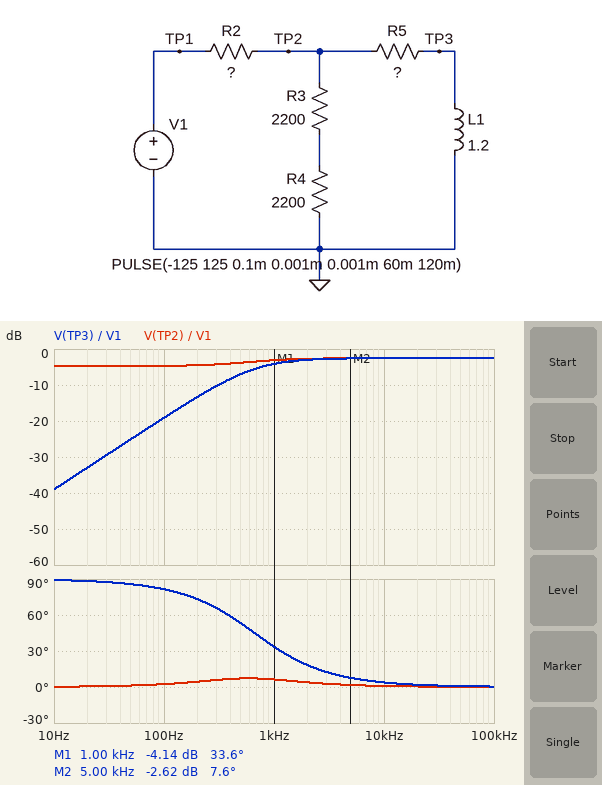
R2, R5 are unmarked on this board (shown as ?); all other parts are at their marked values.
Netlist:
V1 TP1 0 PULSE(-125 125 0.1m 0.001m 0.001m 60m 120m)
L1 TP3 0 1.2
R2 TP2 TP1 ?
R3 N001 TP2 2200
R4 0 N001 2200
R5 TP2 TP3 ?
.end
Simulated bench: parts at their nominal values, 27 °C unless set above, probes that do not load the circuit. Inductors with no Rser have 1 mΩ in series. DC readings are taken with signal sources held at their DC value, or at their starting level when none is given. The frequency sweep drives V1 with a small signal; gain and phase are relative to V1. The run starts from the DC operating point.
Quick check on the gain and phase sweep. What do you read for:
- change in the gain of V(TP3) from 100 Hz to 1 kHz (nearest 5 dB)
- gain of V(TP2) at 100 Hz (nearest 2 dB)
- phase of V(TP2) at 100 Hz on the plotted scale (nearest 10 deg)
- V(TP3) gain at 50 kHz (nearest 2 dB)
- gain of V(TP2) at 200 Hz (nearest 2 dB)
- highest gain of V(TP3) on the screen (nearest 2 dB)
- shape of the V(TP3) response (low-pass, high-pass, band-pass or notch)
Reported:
15 dB
-4 dB
0 deg
-2 dB
-4 dB
-2 dB
high-pass
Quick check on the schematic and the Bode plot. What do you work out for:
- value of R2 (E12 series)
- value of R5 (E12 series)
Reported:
1.5 kΩ
3.9 kΩ
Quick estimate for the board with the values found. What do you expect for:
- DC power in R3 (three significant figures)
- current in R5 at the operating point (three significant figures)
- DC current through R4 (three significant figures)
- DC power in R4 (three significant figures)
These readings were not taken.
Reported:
596 mW
18.6 mA
16.5 mA
596 mW
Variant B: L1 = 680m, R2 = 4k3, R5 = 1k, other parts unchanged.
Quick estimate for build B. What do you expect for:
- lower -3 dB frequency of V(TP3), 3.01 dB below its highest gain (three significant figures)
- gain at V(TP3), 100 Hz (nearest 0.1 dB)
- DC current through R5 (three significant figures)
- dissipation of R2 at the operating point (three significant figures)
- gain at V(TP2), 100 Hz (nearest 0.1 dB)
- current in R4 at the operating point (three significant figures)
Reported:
743 Hz
-23.4 dB
19.9 mA
2.57 W
-15.3 dB
4.53 mA
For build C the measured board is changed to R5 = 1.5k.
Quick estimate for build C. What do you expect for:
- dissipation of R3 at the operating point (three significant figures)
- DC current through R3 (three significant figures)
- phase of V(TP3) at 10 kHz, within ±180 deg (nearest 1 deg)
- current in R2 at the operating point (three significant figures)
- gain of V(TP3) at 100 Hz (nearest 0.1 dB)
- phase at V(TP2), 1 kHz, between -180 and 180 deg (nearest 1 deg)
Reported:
324 mW
12.1 mA
2 deg
47.7 mA
-13.7 dB
8 deg
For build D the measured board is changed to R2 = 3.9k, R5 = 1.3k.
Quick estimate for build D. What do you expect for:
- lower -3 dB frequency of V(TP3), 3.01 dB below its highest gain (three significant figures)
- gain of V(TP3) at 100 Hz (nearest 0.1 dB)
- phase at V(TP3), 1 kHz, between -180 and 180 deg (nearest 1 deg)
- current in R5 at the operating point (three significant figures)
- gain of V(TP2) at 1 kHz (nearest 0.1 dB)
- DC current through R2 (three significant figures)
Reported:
447 Hz
-18.7 dB
24 deg
19.7 mA
-6.2 dB
25.5 mA
